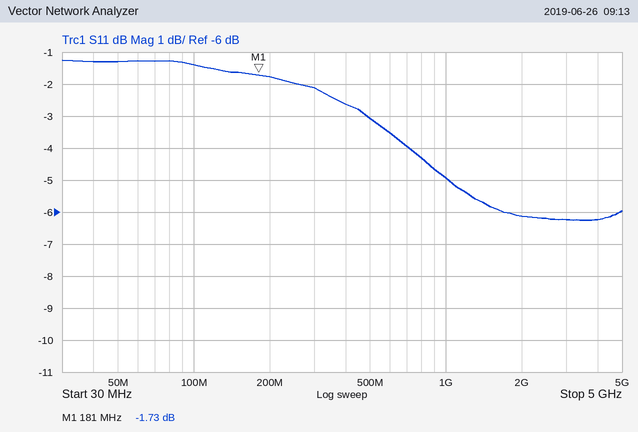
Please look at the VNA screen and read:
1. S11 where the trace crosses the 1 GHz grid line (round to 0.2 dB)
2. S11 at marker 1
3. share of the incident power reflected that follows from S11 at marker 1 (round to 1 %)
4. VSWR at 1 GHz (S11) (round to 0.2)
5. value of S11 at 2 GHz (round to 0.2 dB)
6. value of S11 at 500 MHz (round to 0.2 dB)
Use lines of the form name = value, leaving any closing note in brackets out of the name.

S11 where the trace crosses the 1 GHz grid line = -5.0 dB
S11 at marker 1 = -1.73 dB
share of the incident power reflected that follows from S11 at marker 1 = 67 %
VSWR at 1 GHz (S11) = 3.6
value of S11 at 2 GHz = -6.2 dB
value of S11 at 500 MHz = -3.0 dB
